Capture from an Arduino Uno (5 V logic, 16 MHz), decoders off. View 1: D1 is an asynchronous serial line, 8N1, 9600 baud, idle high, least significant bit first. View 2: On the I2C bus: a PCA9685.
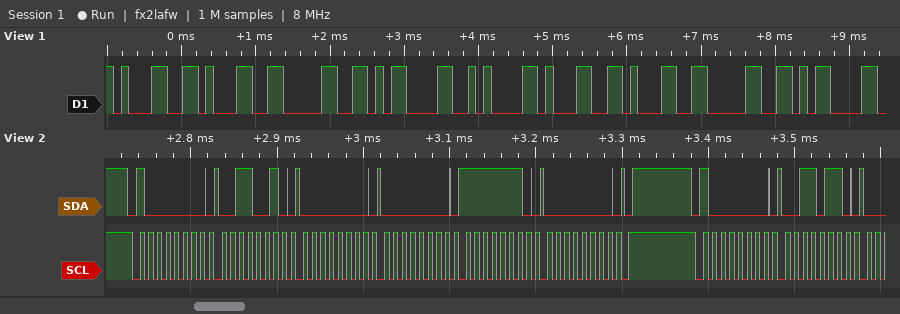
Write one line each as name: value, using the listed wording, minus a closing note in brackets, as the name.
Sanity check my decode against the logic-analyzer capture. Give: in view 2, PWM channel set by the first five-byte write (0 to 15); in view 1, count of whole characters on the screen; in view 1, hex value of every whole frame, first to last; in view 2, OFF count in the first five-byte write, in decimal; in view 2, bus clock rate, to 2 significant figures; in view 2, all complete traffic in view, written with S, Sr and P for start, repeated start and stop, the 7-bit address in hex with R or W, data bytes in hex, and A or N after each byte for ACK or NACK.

in view 2, PWM channel set by the first five-byte write: 11
in view 1, count of whole characters on the screen: 9
in view 1, hex value of every whole frame, first to last: 31 31 30 0D 0A 31 31 30 0D
in view 2, OFF count in the first five-byte write, in decimal: 254
in view 2, bus clock rate, to 2 significant figures: 100 kHz
in view 2, all complete traffic in view, written with S, Sr and P for start, repeated start and stop, the 7-bit address in hex with R or W, data bytes in hex, and A or N after each byte for ACK or NACK: S 40W A 32 A 00 A 00 A FE A 00 A P S 40W A 36 A
